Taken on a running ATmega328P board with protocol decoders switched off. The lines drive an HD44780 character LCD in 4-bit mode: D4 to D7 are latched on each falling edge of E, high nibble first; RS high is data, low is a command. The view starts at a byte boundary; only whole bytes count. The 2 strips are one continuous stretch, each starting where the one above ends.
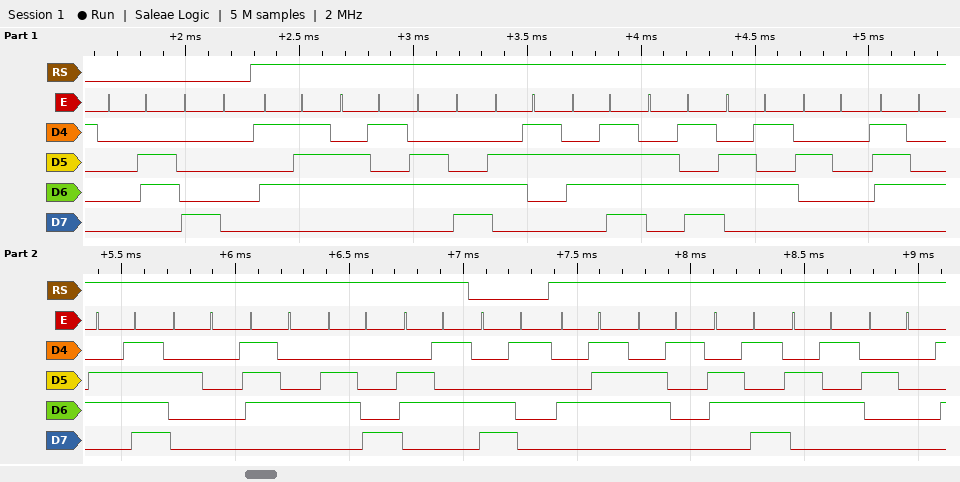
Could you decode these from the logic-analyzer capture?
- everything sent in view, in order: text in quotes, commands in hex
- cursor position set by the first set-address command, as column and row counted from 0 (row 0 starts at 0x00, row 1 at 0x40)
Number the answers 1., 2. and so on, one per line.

1. 0x06 0x80 "Welcome to the" 0xC1 "Game "
2. column 0, row 0
